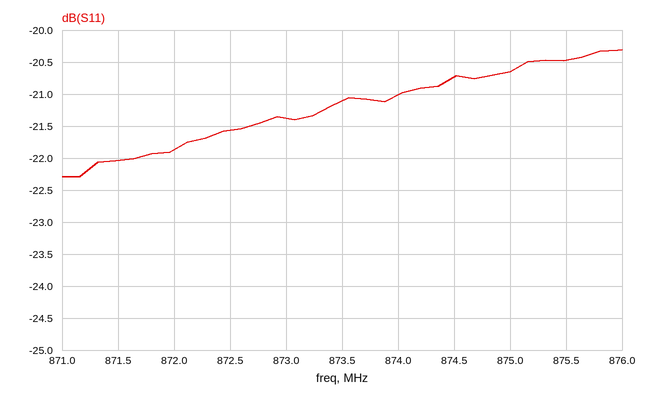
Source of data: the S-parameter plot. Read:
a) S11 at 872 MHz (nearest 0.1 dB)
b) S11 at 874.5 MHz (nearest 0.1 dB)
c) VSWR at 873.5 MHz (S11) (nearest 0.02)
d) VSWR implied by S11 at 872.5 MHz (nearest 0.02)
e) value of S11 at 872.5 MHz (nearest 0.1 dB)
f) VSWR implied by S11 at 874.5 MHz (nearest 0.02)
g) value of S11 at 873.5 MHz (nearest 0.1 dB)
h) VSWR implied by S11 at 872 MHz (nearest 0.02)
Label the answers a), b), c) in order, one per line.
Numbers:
a) -21.9 dB
b) -20.7 dB
c) 1.20
d) 1.18
e) -21.6 dB
f) 1.20
g) -21.1 dB
h) 1.18
